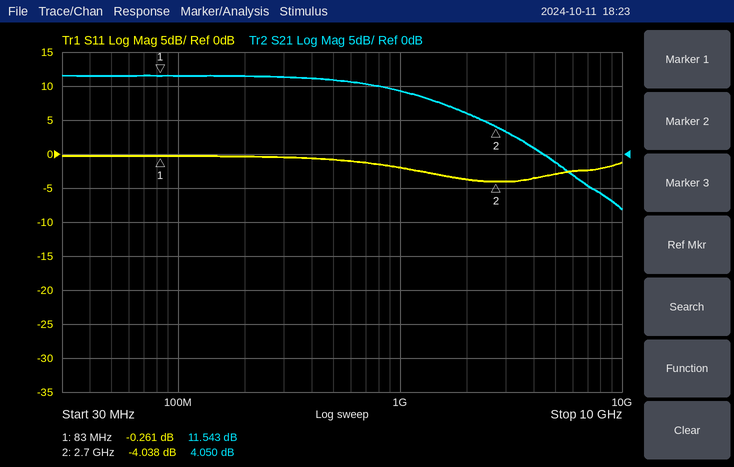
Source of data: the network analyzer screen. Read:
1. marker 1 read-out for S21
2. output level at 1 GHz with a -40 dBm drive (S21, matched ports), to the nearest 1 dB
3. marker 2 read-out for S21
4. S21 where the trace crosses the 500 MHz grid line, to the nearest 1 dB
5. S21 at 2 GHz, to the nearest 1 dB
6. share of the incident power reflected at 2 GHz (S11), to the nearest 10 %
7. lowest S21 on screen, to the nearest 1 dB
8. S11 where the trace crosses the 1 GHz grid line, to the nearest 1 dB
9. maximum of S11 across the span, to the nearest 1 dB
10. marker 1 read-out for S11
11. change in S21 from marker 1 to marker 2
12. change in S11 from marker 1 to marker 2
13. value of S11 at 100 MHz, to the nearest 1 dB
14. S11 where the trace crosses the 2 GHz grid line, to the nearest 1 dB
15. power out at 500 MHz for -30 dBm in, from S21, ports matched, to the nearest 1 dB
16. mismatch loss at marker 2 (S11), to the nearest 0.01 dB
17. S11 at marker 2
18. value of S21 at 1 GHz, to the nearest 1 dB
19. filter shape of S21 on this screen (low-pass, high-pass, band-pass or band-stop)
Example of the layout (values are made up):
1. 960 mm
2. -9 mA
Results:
1. 11.543 dB
2. -31 dBm
3. 4.050 dB
4. 11 dB
5. 6 dB
6. 40 %
7. -8 dB
8. -2 dB
9. 0 dB
10. -0.261 dB
11. -7.493 dB
12. -3.777 dB
13. 0 dB
14. -4 dB
15. -19 dBm
16. 2.18 dB
17. -4.038 dB
18. 9 dB
19. low-pass
